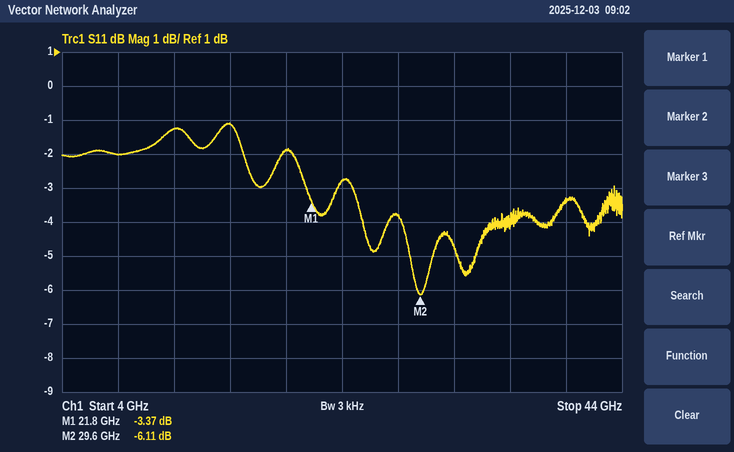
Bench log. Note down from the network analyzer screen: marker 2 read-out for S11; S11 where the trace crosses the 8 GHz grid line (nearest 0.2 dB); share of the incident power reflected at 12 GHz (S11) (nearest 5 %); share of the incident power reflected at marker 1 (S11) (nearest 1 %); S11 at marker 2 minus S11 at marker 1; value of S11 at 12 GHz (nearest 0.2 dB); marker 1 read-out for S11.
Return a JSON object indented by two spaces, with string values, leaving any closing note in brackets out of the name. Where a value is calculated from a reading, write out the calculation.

{
  "marker 2 read-out for S11": "-6.11 dB",
  "S11 where the trace crosses the 8 GHz grid line": "-2.0 dB",
  "share of the incident power reflected at 12 GHz (S11)": "10^(-1.2/10) ≈ 75.9 %, so 75 % to the nearest 5 %",
  "share of the incident power reflected at marker 1 (S11)": "10^(-3.37/10) ≈ 46 %",
  "S11 at marker 2 minus S11 at marker 1": "-6.11 − (-3.37) = -2.74 dB",
  "value of S11 at 12 GHz": "-1.2 dB",
  "marker 1 read-out for S11": "-3.37 dB"
}
